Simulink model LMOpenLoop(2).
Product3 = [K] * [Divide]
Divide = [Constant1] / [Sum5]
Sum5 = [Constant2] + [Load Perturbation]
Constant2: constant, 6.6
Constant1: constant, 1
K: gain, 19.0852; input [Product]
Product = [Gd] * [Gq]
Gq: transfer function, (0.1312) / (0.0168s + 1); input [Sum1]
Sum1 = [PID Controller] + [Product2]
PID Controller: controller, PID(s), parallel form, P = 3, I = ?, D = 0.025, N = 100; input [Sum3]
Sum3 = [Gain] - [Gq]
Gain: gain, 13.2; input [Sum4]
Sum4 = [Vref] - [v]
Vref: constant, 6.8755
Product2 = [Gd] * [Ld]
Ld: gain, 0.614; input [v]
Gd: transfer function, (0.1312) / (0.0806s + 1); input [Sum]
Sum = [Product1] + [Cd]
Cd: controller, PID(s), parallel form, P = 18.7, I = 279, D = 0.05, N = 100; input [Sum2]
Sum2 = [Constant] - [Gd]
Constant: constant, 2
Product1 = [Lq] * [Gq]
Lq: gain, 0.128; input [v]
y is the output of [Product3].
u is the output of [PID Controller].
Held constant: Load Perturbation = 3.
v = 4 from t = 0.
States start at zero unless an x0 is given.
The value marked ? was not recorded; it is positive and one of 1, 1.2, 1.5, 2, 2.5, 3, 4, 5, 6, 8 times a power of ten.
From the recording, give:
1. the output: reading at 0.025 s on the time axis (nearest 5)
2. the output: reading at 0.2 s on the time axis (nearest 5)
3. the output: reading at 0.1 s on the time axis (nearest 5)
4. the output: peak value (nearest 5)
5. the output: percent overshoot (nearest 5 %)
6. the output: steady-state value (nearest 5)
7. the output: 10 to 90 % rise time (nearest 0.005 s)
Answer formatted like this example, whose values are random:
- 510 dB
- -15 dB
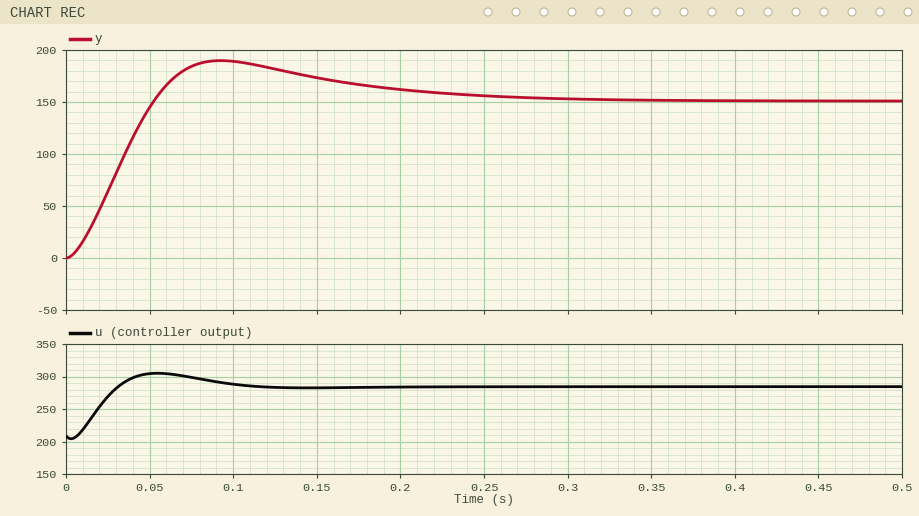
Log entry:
- 65
- 160
- 190
- 190
- 25 %
- 150
- 0.035 s
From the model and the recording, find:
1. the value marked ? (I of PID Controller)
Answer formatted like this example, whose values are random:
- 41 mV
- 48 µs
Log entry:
- 400
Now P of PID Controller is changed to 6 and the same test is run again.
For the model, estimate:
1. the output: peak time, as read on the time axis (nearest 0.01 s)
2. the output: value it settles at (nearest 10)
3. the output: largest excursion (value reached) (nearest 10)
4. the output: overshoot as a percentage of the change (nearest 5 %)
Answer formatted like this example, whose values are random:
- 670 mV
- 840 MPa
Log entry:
- 0.10 s
- 150
- 180
- 20 %
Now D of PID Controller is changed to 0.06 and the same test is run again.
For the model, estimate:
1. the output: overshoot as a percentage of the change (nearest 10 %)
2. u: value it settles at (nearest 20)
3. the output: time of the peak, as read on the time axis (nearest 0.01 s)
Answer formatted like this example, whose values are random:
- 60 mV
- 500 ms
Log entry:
- 30 %
- 280
- 0.10 s
